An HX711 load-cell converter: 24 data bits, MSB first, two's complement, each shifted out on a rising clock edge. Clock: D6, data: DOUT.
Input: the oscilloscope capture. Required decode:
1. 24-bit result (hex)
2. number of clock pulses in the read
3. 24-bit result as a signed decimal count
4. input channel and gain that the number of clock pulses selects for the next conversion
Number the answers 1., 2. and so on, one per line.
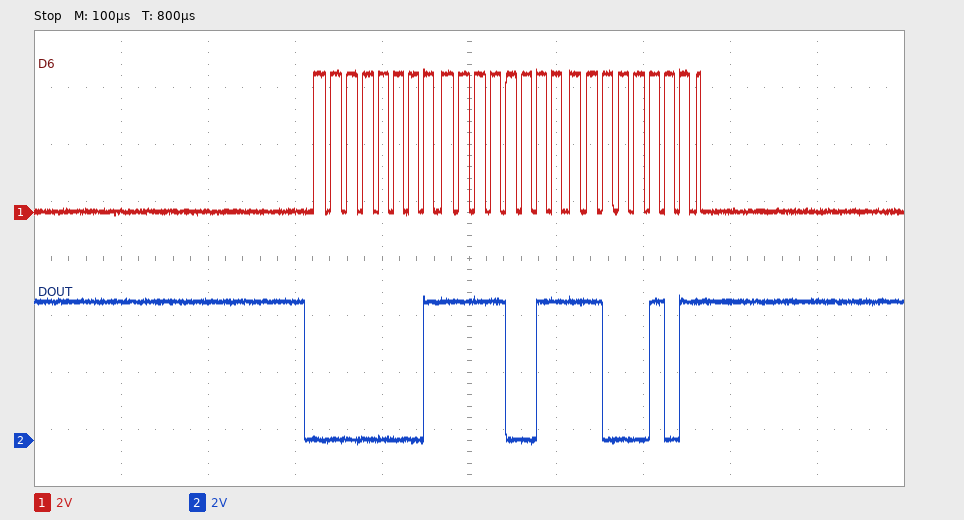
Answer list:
1. 0x01F3C5
2. 25
3. 127941
4. channel A, gain 128
